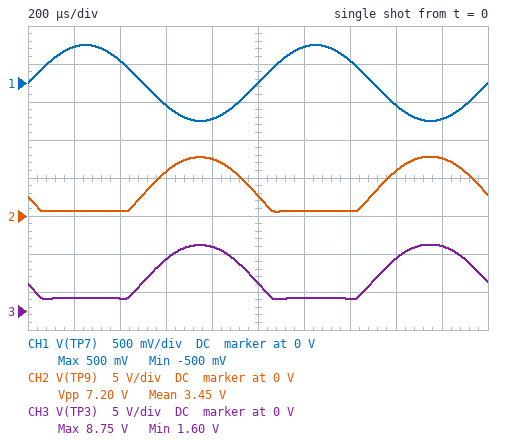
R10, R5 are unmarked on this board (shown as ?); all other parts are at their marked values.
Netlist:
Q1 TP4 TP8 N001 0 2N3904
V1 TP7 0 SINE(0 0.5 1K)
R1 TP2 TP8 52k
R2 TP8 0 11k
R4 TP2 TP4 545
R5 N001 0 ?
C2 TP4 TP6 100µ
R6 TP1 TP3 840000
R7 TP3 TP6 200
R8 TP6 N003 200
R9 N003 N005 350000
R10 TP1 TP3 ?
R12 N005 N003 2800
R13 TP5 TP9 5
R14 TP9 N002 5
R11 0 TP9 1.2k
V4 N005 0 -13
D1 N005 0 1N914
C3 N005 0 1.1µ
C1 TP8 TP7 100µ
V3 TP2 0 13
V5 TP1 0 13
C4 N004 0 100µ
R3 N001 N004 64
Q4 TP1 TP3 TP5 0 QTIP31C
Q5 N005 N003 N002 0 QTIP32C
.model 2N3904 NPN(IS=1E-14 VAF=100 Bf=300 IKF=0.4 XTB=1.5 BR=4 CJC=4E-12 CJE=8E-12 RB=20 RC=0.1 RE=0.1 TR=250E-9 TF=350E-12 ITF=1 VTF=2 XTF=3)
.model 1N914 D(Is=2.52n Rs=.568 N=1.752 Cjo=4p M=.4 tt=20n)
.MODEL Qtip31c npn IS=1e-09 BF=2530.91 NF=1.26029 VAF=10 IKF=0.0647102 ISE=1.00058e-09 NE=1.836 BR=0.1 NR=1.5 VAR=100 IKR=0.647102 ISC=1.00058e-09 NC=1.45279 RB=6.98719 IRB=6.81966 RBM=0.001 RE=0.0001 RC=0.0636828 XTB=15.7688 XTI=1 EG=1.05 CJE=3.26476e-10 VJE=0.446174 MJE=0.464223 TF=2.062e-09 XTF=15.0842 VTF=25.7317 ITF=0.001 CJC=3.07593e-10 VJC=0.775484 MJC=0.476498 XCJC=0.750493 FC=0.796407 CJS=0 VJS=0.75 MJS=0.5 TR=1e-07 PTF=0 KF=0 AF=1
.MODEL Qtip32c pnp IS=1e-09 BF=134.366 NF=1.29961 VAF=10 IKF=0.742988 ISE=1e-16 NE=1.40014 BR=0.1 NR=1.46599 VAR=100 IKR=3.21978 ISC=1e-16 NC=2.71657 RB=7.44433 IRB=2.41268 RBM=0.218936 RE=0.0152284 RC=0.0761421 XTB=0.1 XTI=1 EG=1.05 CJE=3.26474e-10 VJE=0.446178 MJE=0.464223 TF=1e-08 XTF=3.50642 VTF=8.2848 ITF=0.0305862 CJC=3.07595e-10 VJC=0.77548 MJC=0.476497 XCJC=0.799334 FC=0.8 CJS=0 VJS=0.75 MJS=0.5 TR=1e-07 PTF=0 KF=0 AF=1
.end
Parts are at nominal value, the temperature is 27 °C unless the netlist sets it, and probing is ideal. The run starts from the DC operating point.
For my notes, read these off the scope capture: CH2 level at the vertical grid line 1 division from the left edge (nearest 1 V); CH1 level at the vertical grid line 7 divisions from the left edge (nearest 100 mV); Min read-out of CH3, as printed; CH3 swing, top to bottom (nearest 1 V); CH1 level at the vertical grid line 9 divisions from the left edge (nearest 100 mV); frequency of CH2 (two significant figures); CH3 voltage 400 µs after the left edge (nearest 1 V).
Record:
1 V
300 mV
1.60 V
7 V
-500 mV
1.0 kHz
2 V
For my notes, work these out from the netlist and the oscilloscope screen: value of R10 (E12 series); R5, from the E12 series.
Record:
1.8 kΩ
56 Ω
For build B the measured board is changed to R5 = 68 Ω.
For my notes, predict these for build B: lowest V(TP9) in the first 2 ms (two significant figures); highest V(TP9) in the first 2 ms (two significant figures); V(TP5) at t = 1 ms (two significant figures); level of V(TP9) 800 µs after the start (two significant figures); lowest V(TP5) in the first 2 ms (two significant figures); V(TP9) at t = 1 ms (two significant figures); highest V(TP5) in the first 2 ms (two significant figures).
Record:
-250 mV
7.2 V
3.0 V
7.0 V
200 mV
2.6 V
7.6 V
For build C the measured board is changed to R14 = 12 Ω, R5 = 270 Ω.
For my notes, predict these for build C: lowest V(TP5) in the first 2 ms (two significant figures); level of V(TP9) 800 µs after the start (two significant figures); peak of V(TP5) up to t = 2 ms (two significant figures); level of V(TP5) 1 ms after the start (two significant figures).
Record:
23 mV
4.5 V
4.8 V
3.0 V
